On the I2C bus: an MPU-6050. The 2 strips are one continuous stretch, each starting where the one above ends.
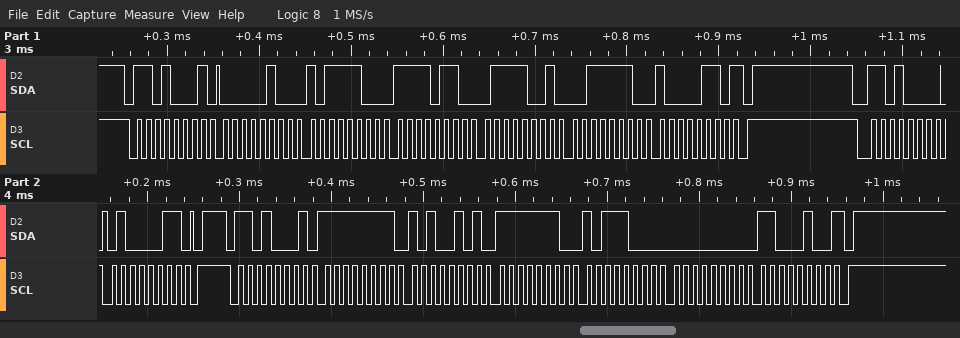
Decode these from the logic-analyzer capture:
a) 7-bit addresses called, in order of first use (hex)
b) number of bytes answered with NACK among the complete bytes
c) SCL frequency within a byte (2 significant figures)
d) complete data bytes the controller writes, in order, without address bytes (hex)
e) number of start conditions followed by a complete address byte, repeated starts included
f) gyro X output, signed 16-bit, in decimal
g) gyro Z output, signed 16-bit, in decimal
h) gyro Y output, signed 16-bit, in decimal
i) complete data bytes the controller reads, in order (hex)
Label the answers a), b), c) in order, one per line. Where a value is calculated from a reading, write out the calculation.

a) 0x68
b) 2
c) 100 kHz
d) 43
e) 3
f) 0xFFA5 = -91
g) 0x00C4 = 196
h) 0xFEB8 = -328
i) 04 BC F6 79 3E 86 FF A5 FE B8 00 C4
